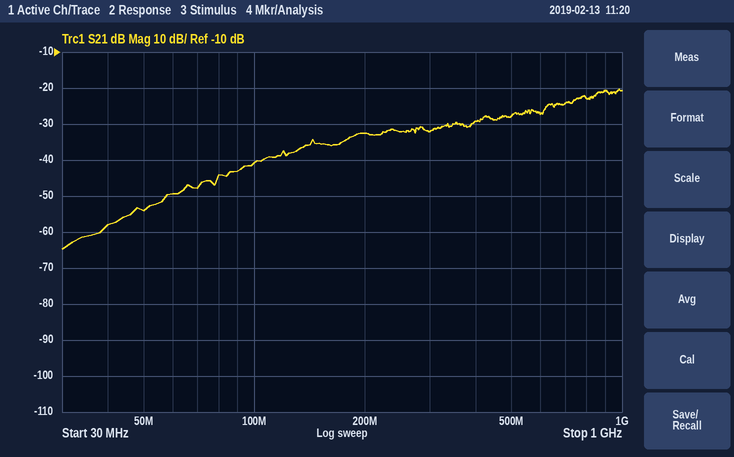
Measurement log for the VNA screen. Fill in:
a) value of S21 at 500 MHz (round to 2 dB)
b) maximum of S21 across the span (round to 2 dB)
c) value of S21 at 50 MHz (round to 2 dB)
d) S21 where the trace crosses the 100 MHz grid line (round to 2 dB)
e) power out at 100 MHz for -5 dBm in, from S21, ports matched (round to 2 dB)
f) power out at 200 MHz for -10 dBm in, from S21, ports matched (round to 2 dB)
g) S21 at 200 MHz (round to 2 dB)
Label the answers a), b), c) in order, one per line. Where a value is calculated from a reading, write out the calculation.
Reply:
a) -28 dB
b) -20 dB
c) -54 dB
d) -40 dB
e) -5 dBm + (-40 dB) = -46 dBm
f) -10 dBm + (-32 dB) = -42 dBm
g) -32 dB
